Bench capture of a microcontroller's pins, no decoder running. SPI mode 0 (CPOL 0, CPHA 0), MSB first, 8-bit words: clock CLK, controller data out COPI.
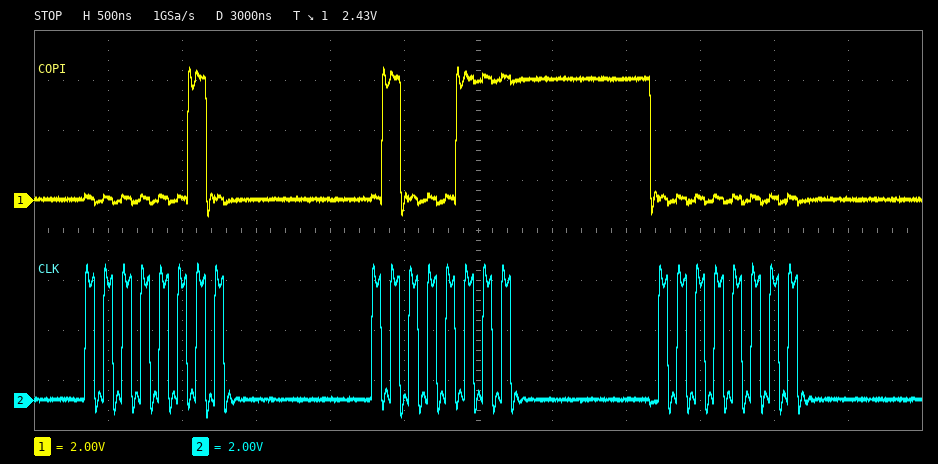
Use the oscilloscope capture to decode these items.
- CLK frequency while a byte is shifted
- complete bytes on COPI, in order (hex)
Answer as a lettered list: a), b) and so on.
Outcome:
a) 8 MHz
b) 02 47 00
